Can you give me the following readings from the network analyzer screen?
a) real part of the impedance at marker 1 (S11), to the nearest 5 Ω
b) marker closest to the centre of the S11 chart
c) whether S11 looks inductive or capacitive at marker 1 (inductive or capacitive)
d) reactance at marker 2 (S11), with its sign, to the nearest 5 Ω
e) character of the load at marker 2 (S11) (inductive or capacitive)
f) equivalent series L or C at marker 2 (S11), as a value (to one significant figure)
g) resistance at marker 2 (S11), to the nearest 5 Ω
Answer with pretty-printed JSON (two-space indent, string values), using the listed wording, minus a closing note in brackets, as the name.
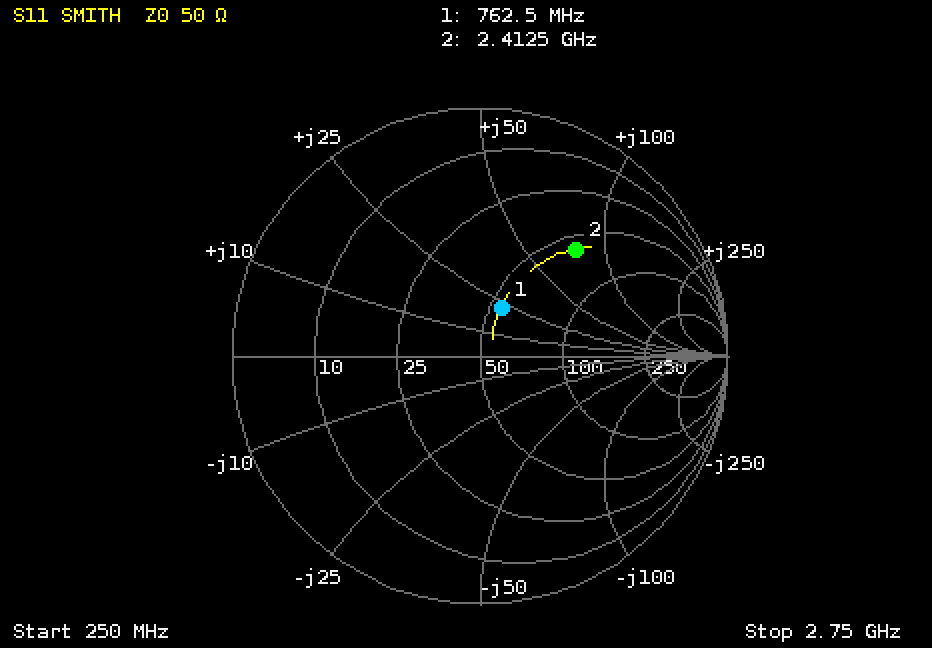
{
  "real part of the impedance at marker 1 (S11), to the nearest 5 Ω": "55 Ω",
  "marker closest to the centre of the S11 chart": "marker 1",
  "whether S11 looks inductive or capacitive at marker 1": "inductive",
  "reactance at marker 2 (S11), with its sign, to the nearest 5 Ω": "+75 Ω",
  "character of the load at marker 2 (S11)": "inductive",
  "equivalent series L or C at marker 2 (S11), as a value": "5 nH",
  "resistance at marker 2 (S11), to the nearest 5 Ω": "60 Ω"
}
